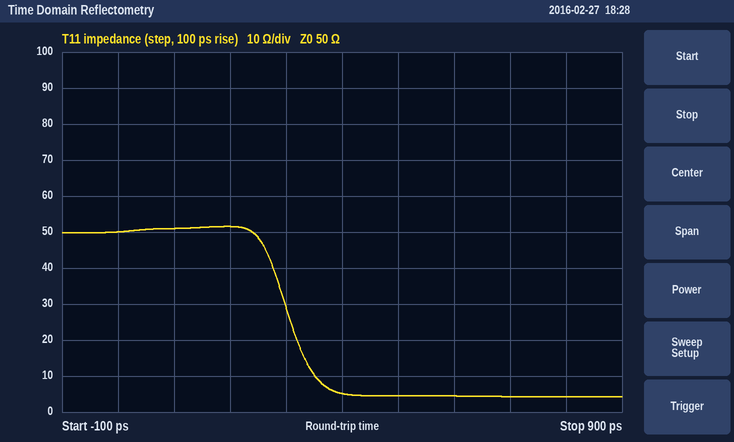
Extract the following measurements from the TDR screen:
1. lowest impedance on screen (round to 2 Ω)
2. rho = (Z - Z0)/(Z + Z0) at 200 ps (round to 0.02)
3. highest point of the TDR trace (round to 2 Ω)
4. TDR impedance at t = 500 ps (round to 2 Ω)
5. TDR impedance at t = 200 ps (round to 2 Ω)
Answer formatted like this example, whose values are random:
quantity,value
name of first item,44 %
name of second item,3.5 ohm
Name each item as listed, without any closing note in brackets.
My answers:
quantity,value
lowest impedance on screen,4 Ω
rho = (Z - Z0)/(Z + Z0) at 200 ps,+0.02
highest point of the TDR trace,52 Ω
TDR impedance at t = 500 ps,4 Ω
TDR impedance at t = 200 ps,52 Ω
